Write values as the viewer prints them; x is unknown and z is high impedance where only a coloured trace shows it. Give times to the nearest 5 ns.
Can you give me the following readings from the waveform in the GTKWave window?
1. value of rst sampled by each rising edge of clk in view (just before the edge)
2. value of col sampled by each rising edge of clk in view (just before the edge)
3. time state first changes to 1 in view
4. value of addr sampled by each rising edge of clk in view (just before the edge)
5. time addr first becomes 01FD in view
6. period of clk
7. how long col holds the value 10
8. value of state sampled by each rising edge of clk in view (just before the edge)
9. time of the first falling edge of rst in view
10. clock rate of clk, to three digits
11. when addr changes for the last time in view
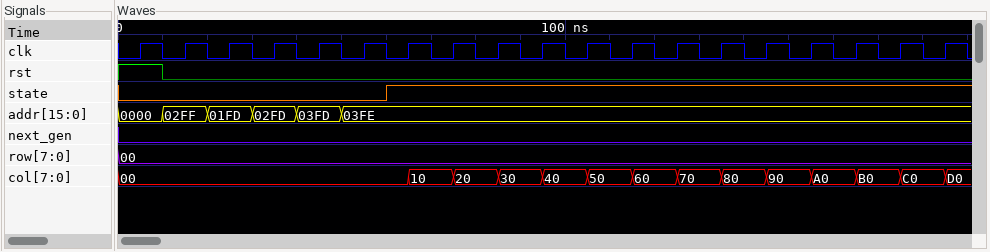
1 0 0 0 0 0 0 0 0 0 0 0 0 0 0 0 0 0 0
00, 00, 00, 00, 00, 00, 00, 10, 20, 30, 40, 50, 60, 70, 80, 90, A0, B0, C0
60 ns
0000, 02FF, 01FD, 02FD, 03FD, 03FE, 03FE, 03FE, 03FE, 03FE, 03FE, 03FE, 03FE, 03FE, 03FE, 03FE, 03FE, 03FE, 03FE
20 ns
10 ns
10 ns
0 0 0 0 0 0 1 1 1 1 1 1 1 1 1 1 1 1 1
10 ns
100 MHz
50 ns
